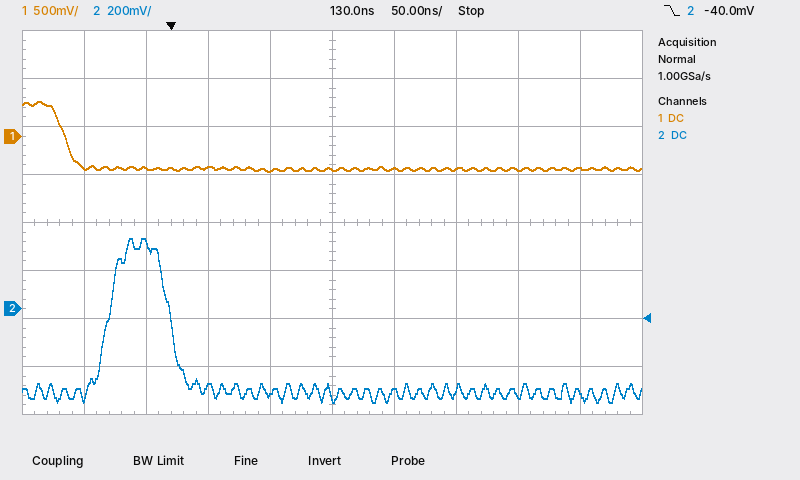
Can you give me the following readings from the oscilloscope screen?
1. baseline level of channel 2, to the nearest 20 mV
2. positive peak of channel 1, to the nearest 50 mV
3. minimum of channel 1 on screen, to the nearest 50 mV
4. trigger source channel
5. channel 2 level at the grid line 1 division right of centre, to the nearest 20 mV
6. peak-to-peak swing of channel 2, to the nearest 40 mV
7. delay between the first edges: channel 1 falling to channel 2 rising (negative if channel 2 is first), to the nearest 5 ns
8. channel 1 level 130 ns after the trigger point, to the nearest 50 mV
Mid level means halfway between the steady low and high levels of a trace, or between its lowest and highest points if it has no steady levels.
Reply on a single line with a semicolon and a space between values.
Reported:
-340 mV; 350 mV; -350 mV; channel 2; -340 mV; 680 mV; +35 ns; -350 mV
